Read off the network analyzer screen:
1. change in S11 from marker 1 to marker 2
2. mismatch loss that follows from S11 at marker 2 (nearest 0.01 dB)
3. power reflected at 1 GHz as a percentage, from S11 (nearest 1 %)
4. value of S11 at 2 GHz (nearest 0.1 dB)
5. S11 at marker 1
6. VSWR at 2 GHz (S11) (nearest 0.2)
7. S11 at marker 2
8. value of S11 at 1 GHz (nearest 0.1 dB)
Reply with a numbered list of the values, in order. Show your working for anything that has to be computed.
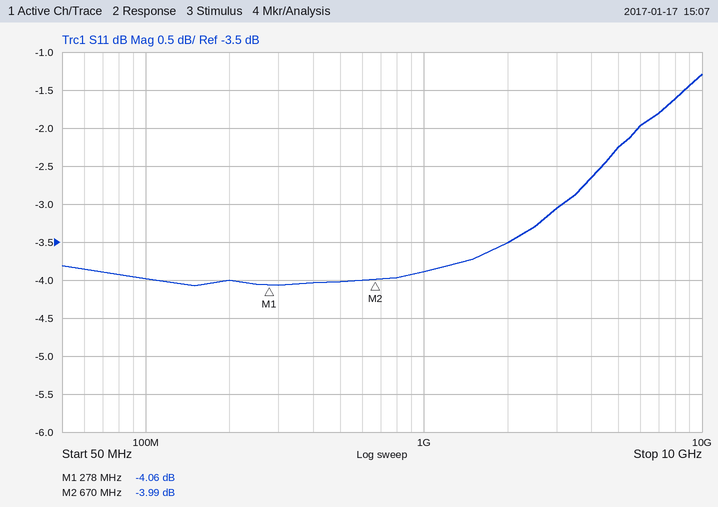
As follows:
1. -3.99 − (-4.06) = 0.07 dB
2. −10 log10(1 − 10^(-3.99/10)) ≈ 2.21 dB
3. 10^(-3.9/10) ≈ 41 %
4. -3.5 dB
5. -4.06 dB
6. |Γ| = 10^(-3.5/20) = 0.6683; VSWR = (1 + 0.6683)/(1 − 0.6683) ≈ 5.0
7. -3.99 dB
8. -3.9 dB
